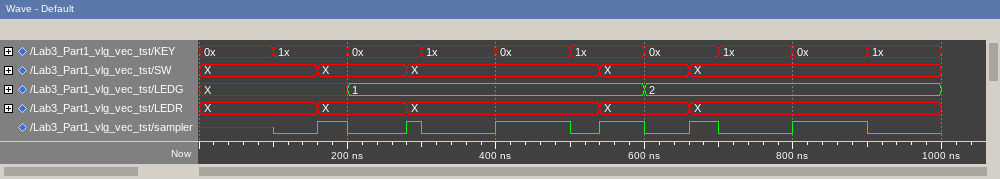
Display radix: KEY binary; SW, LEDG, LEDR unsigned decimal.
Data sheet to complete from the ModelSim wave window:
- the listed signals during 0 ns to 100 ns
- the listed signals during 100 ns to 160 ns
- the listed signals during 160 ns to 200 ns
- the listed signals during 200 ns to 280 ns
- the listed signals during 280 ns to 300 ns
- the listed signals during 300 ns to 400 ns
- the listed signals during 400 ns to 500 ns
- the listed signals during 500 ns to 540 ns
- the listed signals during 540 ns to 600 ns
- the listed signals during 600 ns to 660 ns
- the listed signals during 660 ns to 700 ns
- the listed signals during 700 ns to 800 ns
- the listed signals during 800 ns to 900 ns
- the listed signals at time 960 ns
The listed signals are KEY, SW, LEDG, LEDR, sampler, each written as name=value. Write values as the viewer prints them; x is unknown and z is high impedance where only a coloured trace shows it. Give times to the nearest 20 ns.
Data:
KEY=0x, SW=X, LEDG=X, LEDR=X, sampler=x
KEY=1x, SW=X, LEDG=X, LEDR=X, sampler=0
KEY=1x, SW=X, LEDG=X, LEDR=X, sampler=1
KEY=0x, SW=X, LEDG=1, LEDR=X, sampler=0
KEY=0x, SW=X, LEDG=1, LEDR=X, sampler=1
KEY=1x, SW=X, LEDG=1, LEDR=X, sampler=0
KEY=0x, SW=X, LEDG=1, LEDR=X, sampler=1
KEY=1x, SW=X, LEDG=1, LEDR=X, sampler=0
KEY=1x, SW=X, LEDG=1, LEDR=X, sampler=1
KEY=0x, SW=X, LEDG=2, LEDR=X, sampler=0
KEY=0x, SW=X, LEDG=2, LEDR=X, sampler=1
KEY=1x, SW=X, LEDG=2, LEDR=X, sampler=0
KEY=0x, SW=X, LEDG=2, LEDR=X, sampler=1
KEY=1x, SW=X, LEDG=2, LEDR=X, sampler=0
